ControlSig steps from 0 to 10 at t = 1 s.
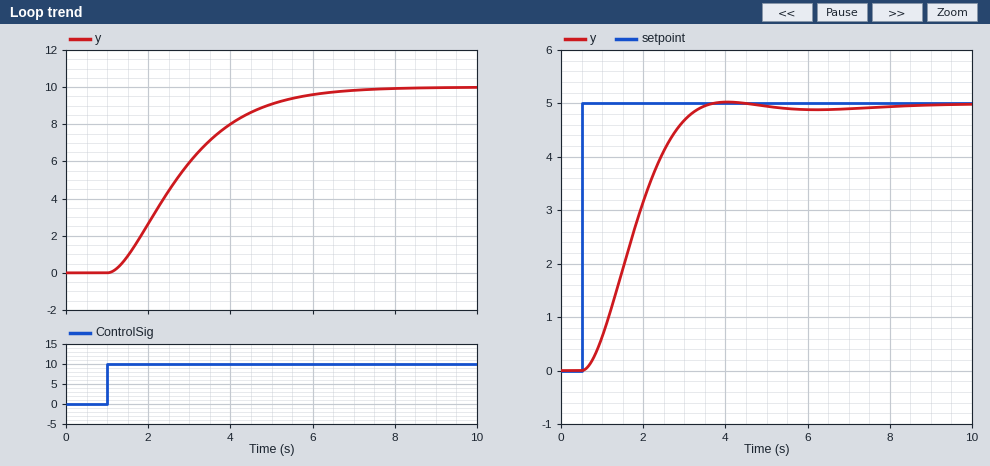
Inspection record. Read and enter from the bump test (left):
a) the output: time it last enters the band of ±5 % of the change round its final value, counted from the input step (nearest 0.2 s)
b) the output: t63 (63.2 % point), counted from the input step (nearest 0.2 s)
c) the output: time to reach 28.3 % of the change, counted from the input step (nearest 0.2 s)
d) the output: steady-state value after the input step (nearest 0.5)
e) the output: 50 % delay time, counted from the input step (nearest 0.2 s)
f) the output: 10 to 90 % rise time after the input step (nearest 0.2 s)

4.8 s
2.2 s
1.0 s
10.0
1.6 s
3.4 s
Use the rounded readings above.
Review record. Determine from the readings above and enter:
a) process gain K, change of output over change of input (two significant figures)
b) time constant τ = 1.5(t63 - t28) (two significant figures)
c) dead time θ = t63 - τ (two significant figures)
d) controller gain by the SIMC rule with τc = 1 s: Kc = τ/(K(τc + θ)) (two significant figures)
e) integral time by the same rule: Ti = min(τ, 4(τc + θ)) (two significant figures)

1.0
1.8 s
0.40 s
1.3
1.8 s
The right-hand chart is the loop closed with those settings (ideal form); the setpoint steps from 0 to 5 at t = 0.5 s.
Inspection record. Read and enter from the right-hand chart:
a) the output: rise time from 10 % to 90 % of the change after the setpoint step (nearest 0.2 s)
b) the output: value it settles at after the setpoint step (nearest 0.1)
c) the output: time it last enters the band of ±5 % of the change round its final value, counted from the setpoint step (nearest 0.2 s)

1.8 s
5.0
2.6 s
